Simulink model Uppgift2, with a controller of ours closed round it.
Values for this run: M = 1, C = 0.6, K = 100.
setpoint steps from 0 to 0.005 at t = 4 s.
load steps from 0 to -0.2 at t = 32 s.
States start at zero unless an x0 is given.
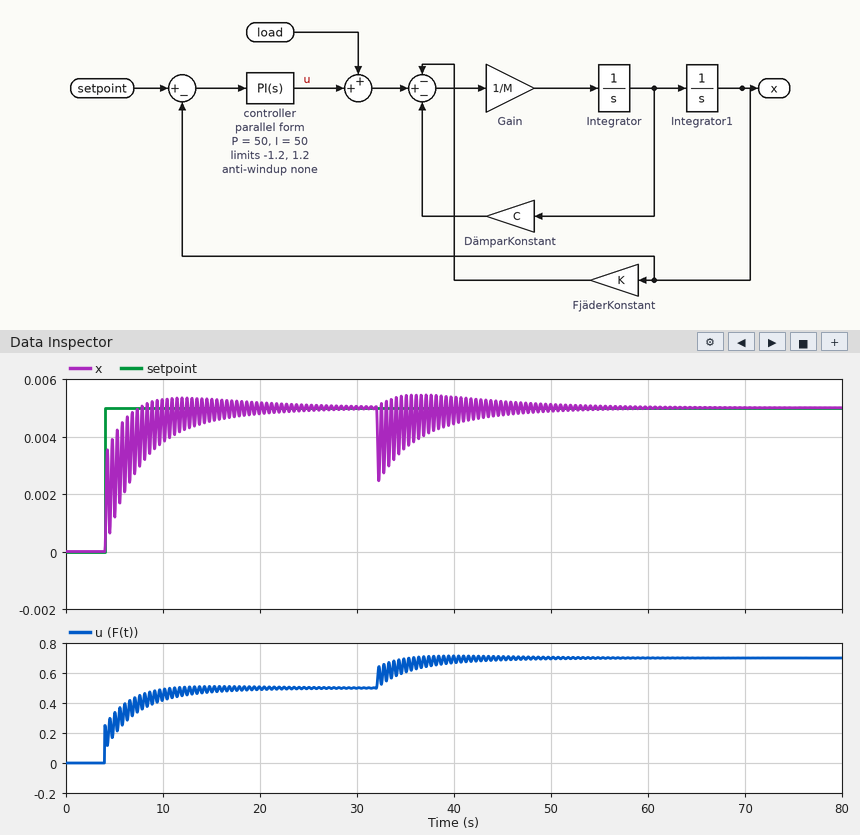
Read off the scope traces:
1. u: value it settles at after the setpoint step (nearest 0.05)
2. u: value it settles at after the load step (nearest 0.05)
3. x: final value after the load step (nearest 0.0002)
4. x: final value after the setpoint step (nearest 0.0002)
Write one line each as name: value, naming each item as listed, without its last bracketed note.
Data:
u: value it settles at after the setpoint step: 0.50
u: value it settles at after the load step: 0.70
x: final value after the load step: 0.0050
x: final value after the setpoint step: 0.0050
